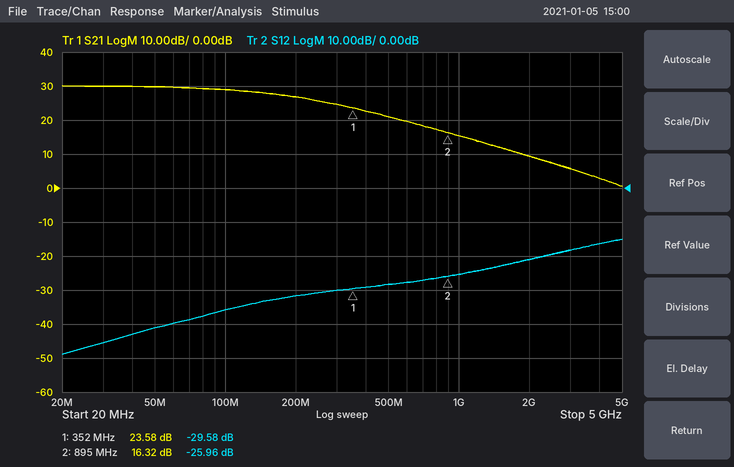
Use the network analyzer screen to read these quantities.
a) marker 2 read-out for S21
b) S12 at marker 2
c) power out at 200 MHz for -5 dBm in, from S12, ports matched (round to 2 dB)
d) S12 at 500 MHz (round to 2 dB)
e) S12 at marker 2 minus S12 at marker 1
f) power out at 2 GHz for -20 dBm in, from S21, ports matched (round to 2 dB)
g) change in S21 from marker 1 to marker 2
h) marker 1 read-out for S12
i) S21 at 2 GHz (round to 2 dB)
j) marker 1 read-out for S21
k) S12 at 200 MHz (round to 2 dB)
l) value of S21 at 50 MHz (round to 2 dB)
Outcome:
16.32 dB
-25.96 dB
-36 dBm
-28 dB
3.62 dB
-10 dBm
-7.26 dB
-29.58 dB
10 dB
23.58 dB
-32 dB
30 dB
